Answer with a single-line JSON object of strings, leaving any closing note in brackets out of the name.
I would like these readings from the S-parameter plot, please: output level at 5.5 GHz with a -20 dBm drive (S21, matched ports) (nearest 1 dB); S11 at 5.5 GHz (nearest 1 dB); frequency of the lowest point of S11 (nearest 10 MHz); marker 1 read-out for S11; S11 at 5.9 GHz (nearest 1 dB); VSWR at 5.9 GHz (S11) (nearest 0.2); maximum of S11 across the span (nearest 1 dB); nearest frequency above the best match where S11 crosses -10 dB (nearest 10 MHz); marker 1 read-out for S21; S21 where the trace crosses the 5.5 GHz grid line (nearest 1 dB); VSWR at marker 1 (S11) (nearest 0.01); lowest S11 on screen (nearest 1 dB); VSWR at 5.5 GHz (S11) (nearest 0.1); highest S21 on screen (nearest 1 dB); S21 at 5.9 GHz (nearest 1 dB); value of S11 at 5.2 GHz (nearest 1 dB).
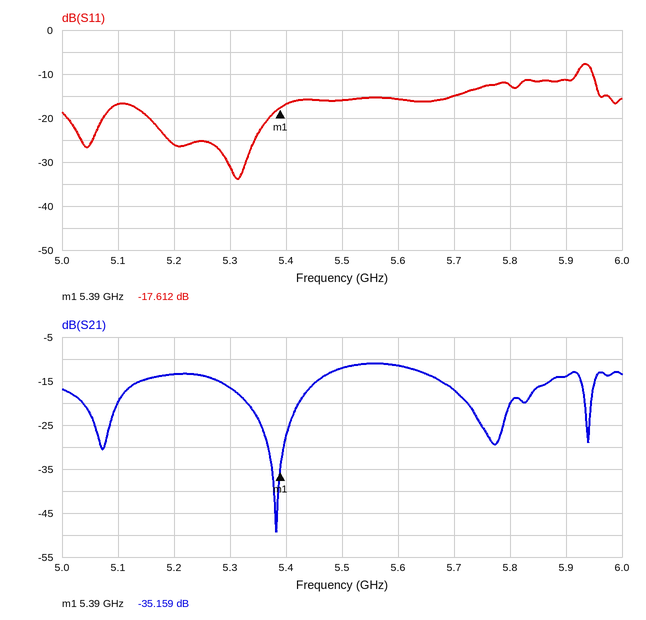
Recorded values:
{"output level at 5.5 GHz with a -20 dBm drive (S21, matched ports)": "-32 dBm", "S11 at 5.5 GHz": "-16 dB", "frequency of the lowest point of S11": "5.31 GHz", "marker 1 read-out for S11": "-17.612 dB", "S11 at 5.9 GHz": "-11 dB", "VSWR at 5.9 GHz (S11)": "1.8", "maximum of S11 across the span": "-8 dB", "nearest frequency above the best match where S11 crosses -10 dB": "5.92 GHz", "marker 1 read-out for S21": "-35.159 dB", "S21 where the trace crosses the 5.5 GHz grid line": "-12 dB", "VSWR at marker 1 (S11)": "1.30", "lowest S11 on screen": "-34 dB", "VSWR at 5.5 GHz (S11)": "1.4", "highest S21 on screen": "-11 dB", "S21 at 5.9 GHz": "-14 dB", "value of S11 at 5.2 GHz": "-26 dB"}
